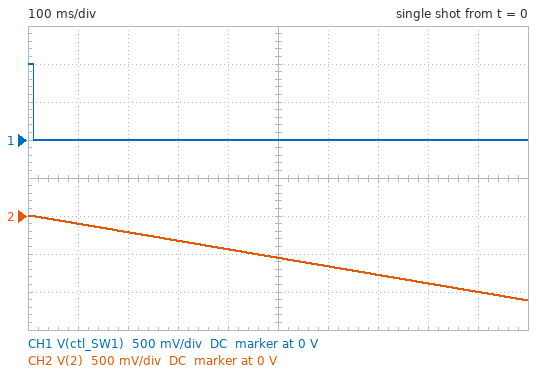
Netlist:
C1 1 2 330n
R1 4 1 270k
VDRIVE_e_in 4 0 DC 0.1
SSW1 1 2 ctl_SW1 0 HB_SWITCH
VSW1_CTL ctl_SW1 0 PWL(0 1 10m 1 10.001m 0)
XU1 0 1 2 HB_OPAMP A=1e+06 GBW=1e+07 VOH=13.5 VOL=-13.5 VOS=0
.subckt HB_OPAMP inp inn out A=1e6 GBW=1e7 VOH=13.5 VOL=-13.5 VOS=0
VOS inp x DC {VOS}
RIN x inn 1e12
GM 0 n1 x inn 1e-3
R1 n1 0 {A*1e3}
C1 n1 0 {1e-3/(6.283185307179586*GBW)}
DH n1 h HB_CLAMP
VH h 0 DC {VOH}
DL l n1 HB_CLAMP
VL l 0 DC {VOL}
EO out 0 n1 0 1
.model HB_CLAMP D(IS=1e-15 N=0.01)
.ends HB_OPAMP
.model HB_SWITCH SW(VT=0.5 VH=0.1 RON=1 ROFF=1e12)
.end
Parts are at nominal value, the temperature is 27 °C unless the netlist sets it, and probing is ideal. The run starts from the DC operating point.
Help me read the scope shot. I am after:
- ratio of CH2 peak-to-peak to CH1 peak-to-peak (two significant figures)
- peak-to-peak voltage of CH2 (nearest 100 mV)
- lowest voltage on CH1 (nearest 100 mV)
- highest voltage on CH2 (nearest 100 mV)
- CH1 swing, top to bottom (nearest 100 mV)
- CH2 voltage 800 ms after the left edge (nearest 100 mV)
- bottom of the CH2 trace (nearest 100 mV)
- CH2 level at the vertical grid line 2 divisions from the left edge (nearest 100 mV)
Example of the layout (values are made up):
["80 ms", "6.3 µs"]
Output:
["1.1", "1.1 V", "0 V", "0 V", "1.0 V", "-900 mV", "-1.1 V", "-200 mV"]
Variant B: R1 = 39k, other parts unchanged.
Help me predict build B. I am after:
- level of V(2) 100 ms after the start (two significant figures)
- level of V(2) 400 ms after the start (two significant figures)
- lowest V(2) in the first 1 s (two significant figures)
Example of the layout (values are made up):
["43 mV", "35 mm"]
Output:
["-700 mV", "-3.0 V", "-7.7 V"]
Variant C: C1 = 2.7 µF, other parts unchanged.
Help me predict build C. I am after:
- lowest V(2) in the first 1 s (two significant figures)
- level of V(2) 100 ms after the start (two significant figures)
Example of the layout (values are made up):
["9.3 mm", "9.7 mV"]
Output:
["-140 mV", "-12 mV"]
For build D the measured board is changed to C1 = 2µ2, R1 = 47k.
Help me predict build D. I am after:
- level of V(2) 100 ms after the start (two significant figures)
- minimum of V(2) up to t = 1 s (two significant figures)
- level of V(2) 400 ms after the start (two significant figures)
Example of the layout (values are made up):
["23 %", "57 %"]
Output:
["-87 mV", "-960 mV", "-380 mV"]
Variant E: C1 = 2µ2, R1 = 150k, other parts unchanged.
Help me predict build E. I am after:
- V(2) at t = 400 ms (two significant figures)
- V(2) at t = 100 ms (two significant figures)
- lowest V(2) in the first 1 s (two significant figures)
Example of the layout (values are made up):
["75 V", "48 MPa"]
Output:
["-120 mV", "-27 mV", "-300 mV"]
